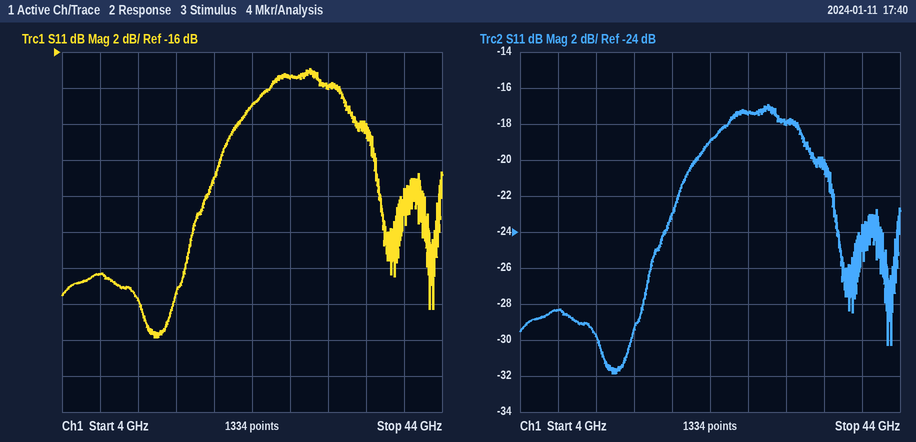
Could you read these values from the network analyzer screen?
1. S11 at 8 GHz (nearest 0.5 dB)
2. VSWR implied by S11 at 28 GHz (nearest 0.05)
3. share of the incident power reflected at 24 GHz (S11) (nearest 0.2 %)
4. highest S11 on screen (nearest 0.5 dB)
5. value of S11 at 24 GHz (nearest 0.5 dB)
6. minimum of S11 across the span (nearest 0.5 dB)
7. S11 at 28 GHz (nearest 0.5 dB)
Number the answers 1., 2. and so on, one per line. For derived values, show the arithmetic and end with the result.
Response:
1. -28.5 dB
2. |Γ| = 10^(-17.5/20) = 0.1334; VSWR = (1 + 0.1334)/(1 − 0.1334) ≈ 1.31, so 1.30 to the nearest 0.05
3. 10^(-19/10) ≈ 1.26 %, so 1.2 % to the nearest 0.2 %
4. -17.0 dB
5. -19.0 dB
6. -32.0 dB
7. -17.5 dB
